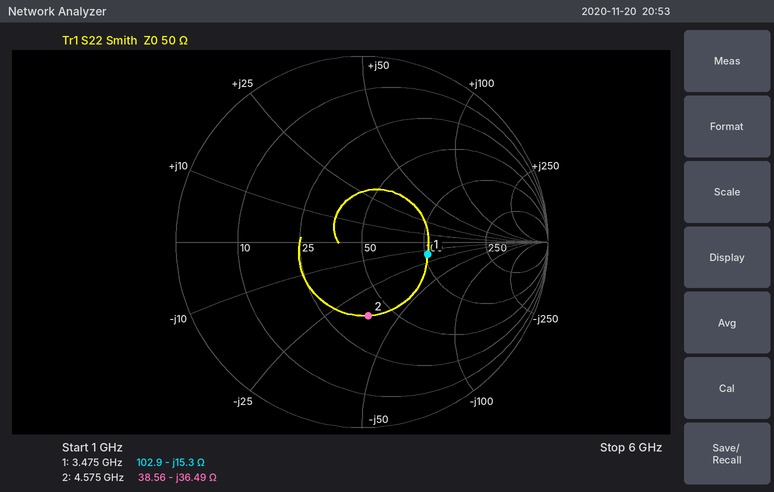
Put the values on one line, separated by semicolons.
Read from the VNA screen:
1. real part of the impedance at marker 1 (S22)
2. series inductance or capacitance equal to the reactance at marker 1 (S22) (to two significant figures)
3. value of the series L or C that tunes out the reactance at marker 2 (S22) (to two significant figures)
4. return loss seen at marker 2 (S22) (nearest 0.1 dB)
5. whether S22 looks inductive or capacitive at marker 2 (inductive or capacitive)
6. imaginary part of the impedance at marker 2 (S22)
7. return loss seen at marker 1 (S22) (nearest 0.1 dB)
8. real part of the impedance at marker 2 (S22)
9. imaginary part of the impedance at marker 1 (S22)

102.9 Ω; 3.0 pF; 1.3 nH; 8.0 dB; capacitive; -36.49 Ω; 8.9 dB; 38.56 Ω; -15.3 Ω
